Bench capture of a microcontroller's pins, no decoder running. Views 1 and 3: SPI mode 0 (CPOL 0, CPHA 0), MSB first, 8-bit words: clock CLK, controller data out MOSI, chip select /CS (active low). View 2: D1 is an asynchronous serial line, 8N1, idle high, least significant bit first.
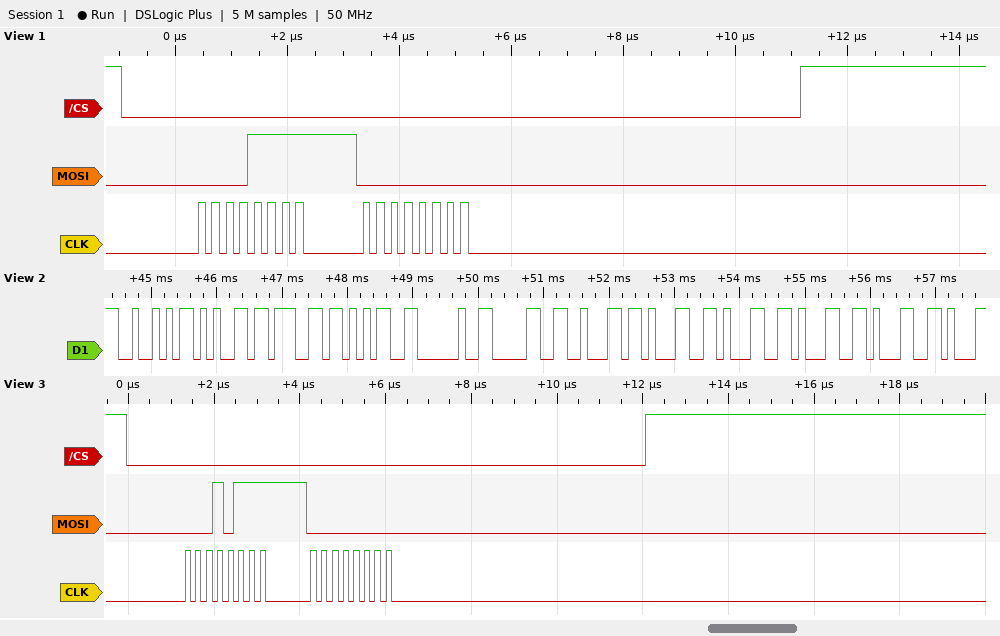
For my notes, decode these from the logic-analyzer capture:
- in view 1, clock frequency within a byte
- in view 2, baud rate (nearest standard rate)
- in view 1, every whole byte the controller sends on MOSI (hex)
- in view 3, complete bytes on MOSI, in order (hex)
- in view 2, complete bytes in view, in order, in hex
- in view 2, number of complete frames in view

4 MHz
9600 baud
0F 00
17 00
52 65 67 35 20 30 62 31 31 31 31
11
